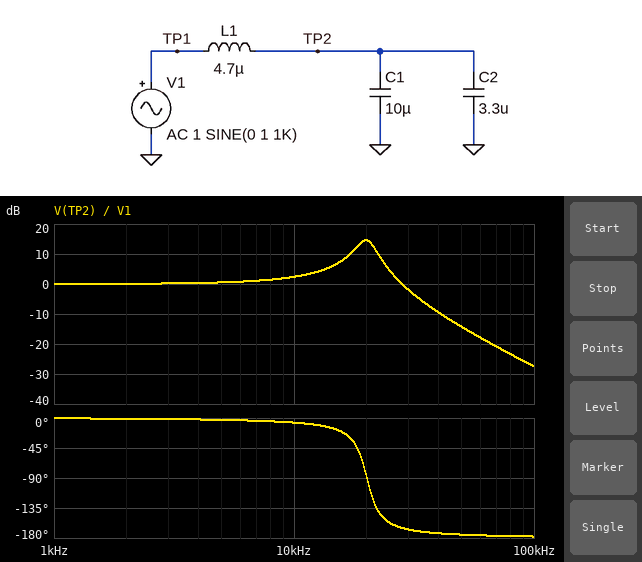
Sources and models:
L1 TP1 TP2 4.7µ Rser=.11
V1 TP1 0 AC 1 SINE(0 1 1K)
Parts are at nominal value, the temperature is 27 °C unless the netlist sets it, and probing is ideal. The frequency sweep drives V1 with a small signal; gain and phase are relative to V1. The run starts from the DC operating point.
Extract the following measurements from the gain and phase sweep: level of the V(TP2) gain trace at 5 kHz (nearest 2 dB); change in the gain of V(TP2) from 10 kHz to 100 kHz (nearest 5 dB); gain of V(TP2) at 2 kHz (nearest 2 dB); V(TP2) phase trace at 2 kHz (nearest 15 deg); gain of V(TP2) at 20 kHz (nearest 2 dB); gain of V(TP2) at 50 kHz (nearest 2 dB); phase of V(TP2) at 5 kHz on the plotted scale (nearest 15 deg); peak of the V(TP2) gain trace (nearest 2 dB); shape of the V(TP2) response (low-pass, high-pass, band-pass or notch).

0 dB
-30 dB
0 dB
0 deg
14 dB
-14 dB
0 deg
14 dB
low-pass
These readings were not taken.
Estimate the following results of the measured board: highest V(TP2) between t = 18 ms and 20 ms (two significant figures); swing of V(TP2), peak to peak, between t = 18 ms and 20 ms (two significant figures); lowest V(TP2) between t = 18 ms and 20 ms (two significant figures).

1.0 V
2.0 V
-1.0 V
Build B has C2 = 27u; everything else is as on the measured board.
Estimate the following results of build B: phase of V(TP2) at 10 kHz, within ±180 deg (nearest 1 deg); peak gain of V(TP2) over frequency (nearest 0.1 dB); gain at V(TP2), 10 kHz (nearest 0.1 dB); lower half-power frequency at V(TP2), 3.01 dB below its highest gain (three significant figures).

-39 deg
10.3 dB
7.9 dB
9.71 kHz
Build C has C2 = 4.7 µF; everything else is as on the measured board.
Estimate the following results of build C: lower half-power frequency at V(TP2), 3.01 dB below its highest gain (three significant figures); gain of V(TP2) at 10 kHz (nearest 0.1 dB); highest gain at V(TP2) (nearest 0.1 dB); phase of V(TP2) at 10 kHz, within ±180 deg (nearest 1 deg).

17.0 kHz
2.7 dB
14.3 dB
-8 deg
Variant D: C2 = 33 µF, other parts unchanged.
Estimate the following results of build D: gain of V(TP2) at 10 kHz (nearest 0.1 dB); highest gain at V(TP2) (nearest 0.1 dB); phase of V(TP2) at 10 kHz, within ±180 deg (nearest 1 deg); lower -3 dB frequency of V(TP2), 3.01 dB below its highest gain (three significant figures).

8.9 dB
9.7 dB
-56 deg
8.79 kHz
